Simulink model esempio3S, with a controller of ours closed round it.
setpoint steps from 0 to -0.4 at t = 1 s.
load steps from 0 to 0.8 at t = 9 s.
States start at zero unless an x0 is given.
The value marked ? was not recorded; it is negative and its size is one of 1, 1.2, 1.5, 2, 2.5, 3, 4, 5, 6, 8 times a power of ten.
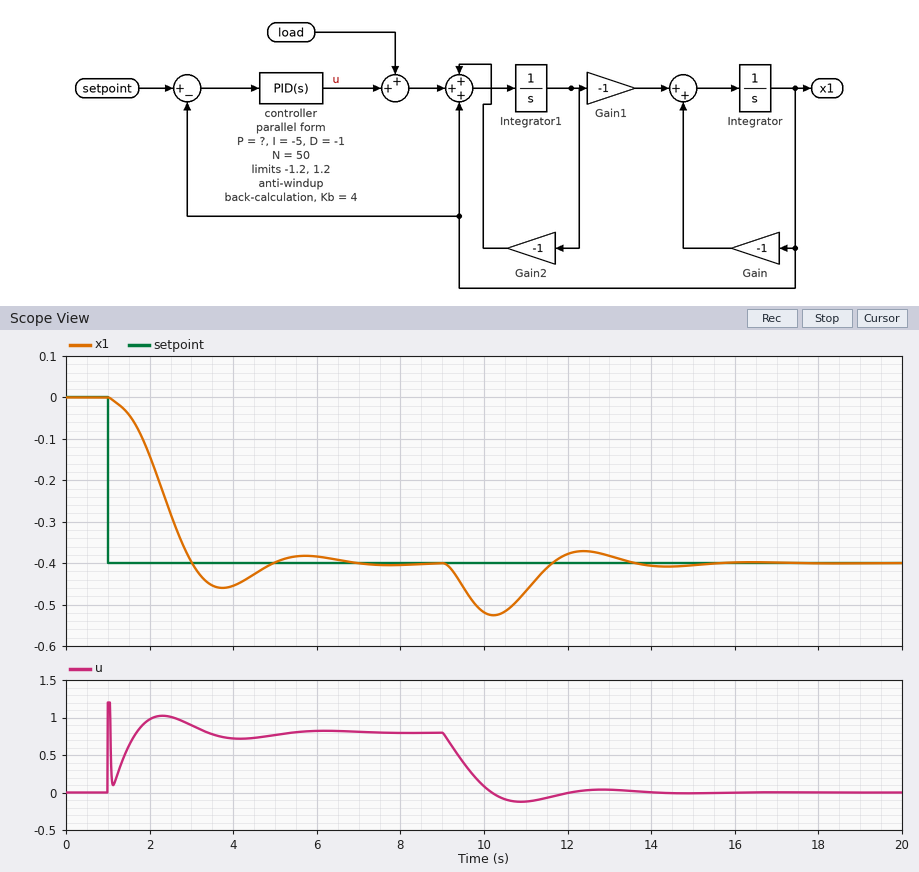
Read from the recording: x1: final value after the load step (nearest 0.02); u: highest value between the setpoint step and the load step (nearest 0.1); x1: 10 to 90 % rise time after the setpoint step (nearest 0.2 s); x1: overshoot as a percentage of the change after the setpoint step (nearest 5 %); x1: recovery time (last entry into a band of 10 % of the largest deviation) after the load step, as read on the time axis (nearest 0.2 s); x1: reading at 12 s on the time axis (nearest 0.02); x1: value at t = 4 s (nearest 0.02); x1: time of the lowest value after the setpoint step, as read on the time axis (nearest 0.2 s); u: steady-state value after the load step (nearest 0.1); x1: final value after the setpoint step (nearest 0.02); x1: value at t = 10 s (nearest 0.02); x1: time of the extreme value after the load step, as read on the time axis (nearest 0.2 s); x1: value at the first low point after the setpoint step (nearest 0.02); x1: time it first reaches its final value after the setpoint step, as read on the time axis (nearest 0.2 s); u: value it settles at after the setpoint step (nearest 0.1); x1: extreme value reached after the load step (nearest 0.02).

-0.40
1.2
1.4 s
15 %
13.2 s
-0.38
-0.46
3.8 s
0.0
-0.40
-0.52
10.2 s
-0.46
3.0 s
0.8
-0.52
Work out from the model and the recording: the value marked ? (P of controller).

-3
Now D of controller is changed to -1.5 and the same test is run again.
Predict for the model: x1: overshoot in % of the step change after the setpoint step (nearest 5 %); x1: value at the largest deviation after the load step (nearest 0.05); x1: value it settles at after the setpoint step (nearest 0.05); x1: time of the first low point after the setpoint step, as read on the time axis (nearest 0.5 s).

20 %
-0.50
-0.40
4.0 s
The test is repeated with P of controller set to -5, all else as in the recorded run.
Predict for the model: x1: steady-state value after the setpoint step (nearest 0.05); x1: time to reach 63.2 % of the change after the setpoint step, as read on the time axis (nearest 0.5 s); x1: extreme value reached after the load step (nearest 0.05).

-0.40
2.0 s
-0.50
